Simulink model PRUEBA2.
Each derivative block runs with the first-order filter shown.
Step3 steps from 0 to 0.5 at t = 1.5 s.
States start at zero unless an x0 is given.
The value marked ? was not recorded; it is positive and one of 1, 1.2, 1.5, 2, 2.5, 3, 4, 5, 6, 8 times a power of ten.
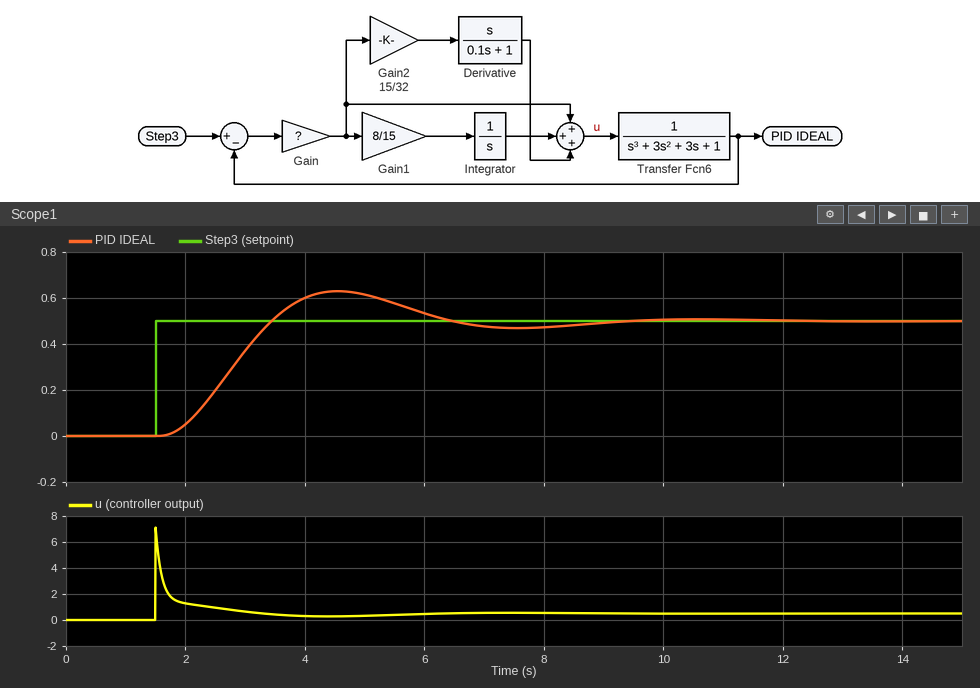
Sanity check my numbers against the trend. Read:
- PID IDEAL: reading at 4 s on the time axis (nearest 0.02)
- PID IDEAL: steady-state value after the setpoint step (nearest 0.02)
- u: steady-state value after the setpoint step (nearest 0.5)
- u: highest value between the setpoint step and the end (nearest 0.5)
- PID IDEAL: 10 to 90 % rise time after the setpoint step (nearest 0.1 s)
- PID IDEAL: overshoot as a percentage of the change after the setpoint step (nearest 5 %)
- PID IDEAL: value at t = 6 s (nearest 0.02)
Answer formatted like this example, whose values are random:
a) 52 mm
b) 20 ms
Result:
a) 0.60
b) 0.50
c) 0.5
d) 7.0
e) 1.3 s
f) 25 %
g) 0.54
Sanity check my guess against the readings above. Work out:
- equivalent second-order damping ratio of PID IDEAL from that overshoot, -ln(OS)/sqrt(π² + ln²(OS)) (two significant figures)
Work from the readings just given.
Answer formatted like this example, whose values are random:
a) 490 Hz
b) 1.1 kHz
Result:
a) 0.40
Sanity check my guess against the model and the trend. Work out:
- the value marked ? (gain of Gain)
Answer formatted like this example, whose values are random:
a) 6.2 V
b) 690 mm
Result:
a) 2.5
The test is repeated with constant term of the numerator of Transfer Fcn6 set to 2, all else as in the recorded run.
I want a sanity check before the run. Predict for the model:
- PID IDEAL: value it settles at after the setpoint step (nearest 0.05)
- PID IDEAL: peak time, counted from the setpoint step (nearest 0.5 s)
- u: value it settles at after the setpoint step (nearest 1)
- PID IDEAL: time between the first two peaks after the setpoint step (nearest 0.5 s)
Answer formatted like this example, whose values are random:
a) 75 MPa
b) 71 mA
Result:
a) 0.50
b) 2.0 s
c) 0
d) 4.0 s
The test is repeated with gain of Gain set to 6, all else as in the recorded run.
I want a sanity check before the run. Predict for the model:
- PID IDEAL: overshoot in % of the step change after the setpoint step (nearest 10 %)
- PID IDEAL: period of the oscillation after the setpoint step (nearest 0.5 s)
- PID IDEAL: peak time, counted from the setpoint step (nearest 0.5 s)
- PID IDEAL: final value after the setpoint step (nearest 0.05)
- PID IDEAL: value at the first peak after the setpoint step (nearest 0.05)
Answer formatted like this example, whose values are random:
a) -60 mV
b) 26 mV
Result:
a) 50 %
b) 3.5 s
c) 2.0 s
d) 0.50
e) 0.75
